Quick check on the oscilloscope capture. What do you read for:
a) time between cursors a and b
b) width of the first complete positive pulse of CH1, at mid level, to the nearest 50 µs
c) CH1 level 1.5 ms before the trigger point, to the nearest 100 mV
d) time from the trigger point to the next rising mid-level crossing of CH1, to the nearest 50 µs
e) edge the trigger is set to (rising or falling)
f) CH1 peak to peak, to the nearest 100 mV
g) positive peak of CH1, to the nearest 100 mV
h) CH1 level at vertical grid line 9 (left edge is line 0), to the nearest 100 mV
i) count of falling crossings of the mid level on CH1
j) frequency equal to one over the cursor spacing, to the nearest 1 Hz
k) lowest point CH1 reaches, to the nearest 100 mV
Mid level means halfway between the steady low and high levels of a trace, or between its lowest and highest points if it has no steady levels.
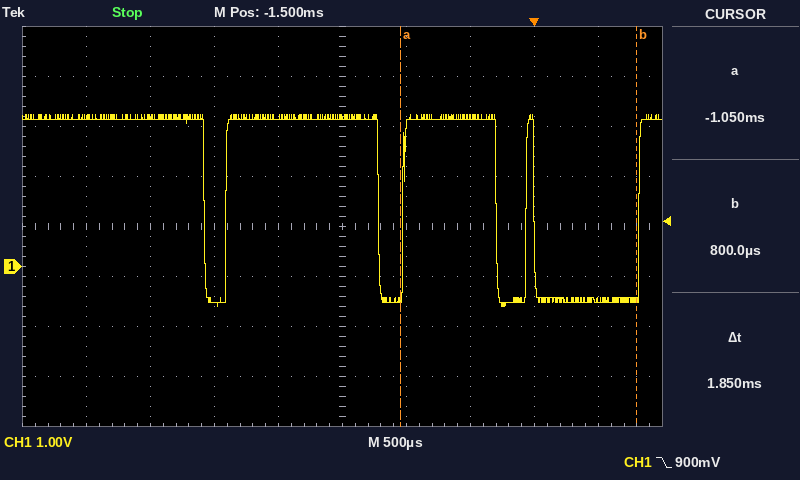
1.85 ms
1.20 ms
3.0 V
800 µs
falling
3.8 V
3.0 V
-700 mV
4
541 Hz
-800 mV
